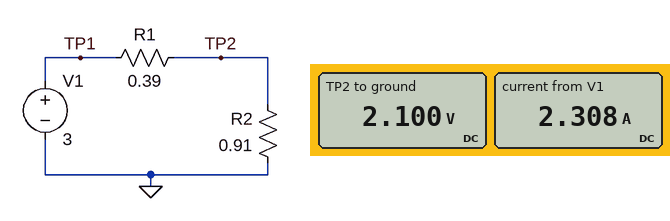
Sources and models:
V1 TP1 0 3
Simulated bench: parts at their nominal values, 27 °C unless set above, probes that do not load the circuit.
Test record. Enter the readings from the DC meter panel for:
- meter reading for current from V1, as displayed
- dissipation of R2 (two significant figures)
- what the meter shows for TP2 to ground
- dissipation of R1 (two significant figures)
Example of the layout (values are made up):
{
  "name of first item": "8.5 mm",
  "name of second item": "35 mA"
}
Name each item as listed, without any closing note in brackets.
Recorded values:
{
  "meter reading for current from V1, as displayed": "2.308 A",
  "dissipation of R2": "4.8 W",
  "what the meter shows for TP2 to ground": "2.100 V",
  "dissipation of R1": "2.1 W"
}
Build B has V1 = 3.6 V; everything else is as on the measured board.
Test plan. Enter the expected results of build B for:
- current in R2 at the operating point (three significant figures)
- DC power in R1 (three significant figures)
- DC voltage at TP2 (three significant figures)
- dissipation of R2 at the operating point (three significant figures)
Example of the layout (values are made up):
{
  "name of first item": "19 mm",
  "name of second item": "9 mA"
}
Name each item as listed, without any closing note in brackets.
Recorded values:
{
  "current in R2 at the operating point": "2.77 A",
  "DC power in R1": "2.99 W",
  "DC voltage at TP2": "2.52 V",
  "dissipation of R2 at the operating point": "6.98 W"
}
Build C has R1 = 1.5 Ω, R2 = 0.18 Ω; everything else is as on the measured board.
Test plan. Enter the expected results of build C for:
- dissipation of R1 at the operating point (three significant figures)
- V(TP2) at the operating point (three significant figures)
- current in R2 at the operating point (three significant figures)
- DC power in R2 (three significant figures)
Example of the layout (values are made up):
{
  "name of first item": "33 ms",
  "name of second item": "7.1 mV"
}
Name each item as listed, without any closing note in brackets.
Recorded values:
{
  "dissipation of R1 at the operating point": "4.78 W",
  "V(TP2) at the operating point": "321 mV",
  "current in R2 at the operating point": "1.79 A",
  "DC power in R2": "574 mW"
}
